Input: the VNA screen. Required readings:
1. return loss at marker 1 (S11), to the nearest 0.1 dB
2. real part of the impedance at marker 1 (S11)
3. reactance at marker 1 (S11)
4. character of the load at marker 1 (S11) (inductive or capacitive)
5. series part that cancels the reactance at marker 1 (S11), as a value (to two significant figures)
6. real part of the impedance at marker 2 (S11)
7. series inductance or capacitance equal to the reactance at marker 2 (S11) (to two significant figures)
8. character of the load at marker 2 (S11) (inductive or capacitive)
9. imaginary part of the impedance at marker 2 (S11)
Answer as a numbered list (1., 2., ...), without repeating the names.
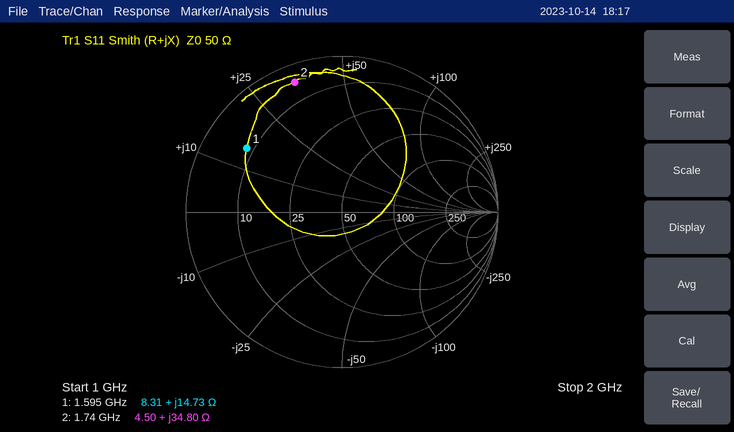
1. 2.7 dB
2. 8.31 Ω
3. +14.73 Ω
4. inductive
5. 6.8 pF
6. 4.50 Ω
7. 3.2 nH
8. inductive
9. +34.80 Ω
